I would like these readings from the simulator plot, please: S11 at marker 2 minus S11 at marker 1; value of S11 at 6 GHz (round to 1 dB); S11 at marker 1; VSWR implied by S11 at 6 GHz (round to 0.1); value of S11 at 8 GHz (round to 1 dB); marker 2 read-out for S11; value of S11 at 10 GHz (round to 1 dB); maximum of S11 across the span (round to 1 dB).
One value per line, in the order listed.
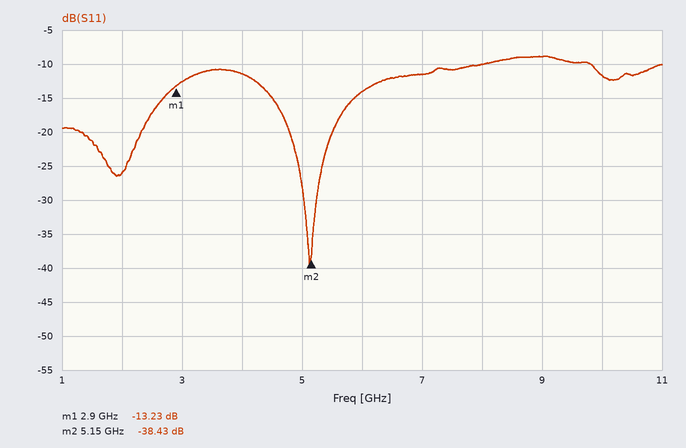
-25.20 dB
-14 dB
-13.23 dB
1.5
-10 dB
-38.43 dB
-12 dB
-9 dB
